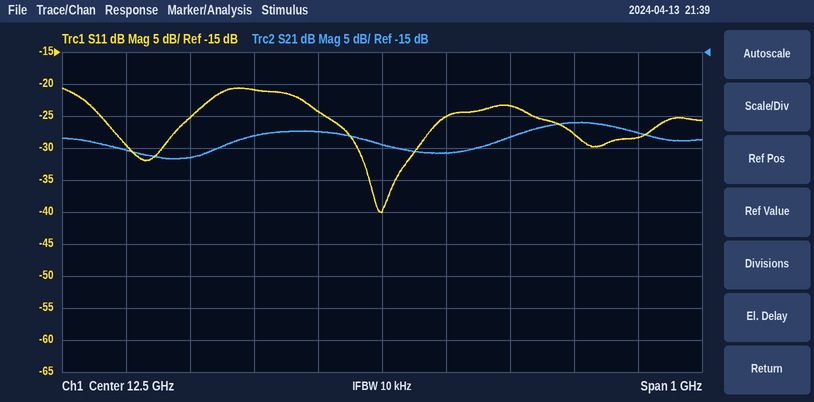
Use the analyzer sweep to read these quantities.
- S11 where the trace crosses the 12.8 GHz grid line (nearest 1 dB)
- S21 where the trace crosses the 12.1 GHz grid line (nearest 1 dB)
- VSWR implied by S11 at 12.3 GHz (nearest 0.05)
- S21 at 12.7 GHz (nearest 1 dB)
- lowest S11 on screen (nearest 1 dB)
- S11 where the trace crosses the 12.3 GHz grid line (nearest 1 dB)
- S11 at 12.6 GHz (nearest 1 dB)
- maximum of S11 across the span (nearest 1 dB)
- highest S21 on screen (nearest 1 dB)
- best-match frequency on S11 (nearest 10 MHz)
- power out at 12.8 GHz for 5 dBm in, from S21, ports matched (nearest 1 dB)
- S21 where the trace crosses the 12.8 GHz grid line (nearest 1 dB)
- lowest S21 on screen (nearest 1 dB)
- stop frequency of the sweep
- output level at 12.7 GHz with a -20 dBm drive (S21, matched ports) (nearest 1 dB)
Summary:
-28 dB
-30 dB
1.20
-28 dB
-40 dB
-21 dB
-25 dB
-21 dB
-26 dB
12.50 GHz
-21 dBm
-26 dB
-32 dB
13 GHz
-48 dBm
